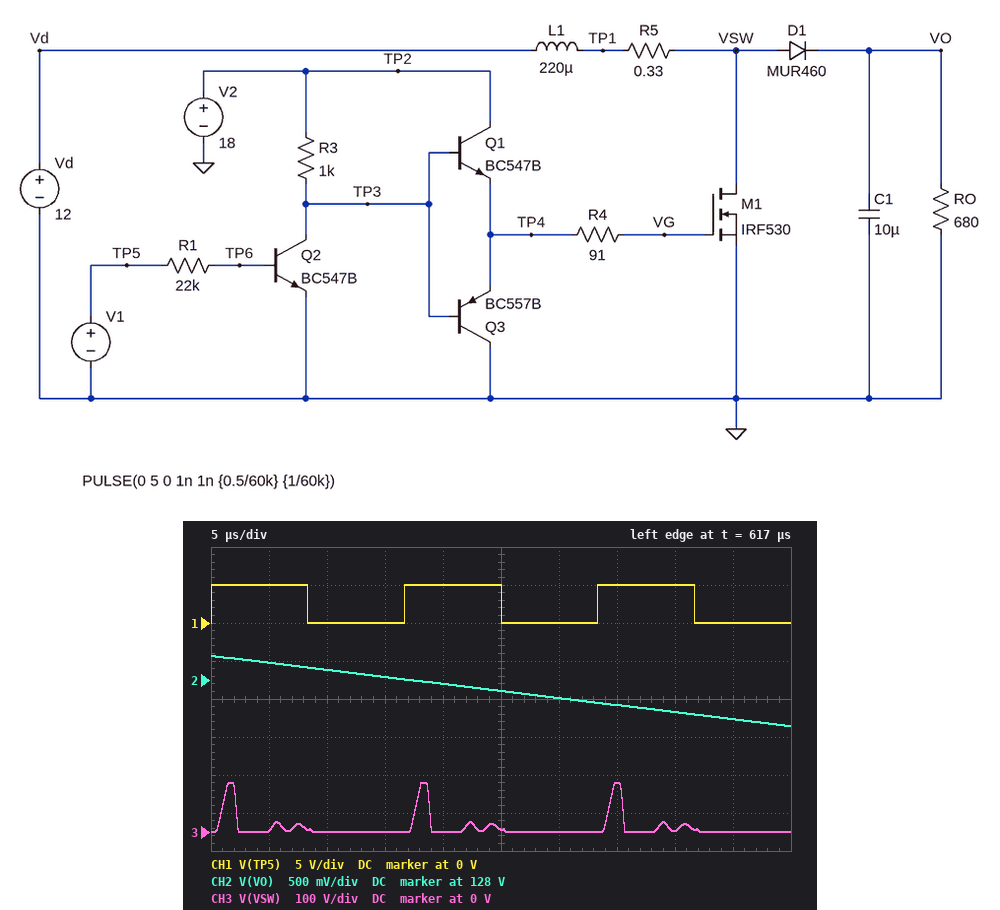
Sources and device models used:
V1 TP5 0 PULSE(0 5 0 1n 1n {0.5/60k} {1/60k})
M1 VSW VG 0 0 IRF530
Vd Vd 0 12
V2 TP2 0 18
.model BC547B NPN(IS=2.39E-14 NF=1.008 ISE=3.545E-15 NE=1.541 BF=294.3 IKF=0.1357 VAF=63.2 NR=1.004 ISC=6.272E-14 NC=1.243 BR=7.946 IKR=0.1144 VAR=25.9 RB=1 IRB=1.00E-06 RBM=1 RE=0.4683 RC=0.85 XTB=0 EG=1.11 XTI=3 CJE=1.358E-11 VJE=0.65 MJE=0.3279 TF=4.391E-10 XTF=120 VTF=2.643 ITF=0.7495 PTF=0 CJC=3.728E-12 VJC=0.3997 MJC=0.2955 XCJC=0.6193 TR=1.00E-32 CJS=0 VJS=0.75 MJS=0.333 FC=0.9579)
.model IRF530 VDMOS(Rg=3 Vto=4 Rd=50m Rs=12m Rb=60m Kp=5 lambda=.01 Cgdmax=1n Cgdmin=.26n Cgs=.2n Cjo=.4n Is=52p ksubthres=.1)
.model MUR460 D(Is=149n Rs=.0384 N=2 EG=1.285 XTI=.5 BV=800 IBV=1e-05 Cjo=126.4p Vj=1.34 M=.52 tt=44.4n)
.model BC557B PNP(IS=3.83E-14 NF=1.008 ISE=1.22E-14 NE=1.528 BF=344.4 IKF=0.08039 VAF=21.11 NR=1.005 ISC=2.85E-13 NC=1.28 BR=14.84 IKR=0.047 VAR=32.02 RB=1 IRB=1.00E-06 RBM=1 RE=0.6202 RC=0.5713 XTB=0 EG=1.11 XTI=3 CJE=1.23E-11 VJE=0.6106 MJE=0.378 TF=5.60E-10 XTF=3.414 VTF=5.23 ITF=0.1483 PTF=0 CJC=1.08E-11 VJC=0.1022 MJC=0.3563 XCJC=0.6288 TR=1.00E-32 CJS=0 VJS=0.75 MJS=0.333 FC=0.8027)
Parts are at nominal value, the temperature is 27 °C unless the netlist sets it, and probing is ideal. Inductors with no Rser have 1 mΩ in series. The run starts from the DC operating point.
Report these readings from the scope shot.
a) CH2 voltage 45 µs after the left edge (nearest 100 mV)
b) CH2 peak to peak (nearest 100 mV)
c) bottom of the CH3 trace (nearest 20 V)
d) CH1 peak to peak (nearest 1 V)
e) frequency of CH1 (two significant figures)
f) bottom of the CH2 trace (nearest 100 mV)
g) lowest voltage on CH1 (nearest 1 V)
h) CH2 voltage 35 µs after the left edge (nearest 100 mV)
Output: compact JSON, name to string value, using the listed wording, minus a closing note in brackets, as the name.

{"CH2 voltage 45 µs after the left edge": "127.5 V", "CH2 peak to peak": "900 mV", "bottom of the CH3 trace": "0 V", "CH1 peak to peak": "5 V", "frequency of CH1": "60 kHz", "bottom of the CH2 trace": "127.4 V", "lowest voltage on CH1": "0 V", "CH2 voltage 35 µs after the left edge": "127.7 V"}
